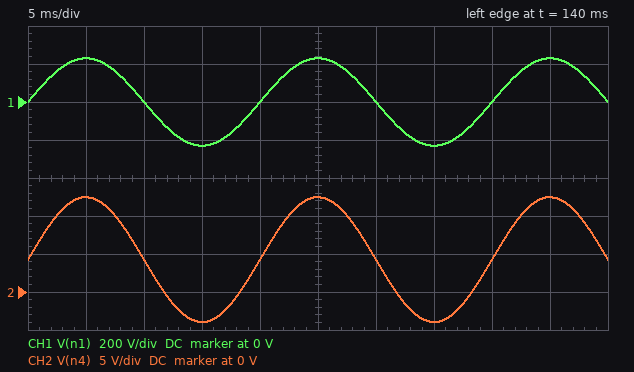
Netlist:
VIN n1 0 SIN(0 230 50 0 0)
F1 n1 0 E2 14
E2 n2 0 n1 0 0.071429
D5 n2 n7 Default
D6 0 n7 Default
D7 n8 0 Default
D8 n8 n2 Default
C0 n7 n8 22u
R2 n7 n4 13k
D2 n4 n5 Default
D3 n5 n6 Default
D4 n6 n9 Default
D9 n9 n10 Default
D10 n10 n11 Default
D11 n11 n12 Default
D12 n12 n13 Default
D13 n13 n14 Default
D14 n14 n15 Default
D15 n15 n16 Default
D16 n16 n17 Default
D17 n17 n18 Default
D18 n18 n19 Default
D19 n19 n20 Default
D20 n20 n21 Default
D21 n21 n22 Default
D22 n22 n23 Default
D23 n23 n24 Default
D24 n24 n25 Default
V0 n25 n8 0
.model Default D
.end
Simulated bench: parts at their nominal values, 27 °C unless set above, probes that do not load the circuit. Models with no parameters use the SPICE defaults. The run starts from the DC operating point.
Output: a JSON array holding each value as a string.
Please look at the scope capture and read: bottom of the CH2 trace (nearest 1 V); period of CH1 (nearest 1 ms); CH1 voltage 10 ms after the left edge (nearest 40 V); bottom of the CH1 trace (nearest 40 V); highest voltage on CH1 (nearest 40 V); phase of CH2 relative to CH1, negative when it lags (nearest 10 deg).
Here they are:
["-4 V", "20 ms", "0 V", "-240 V", "240 V", "0 deg"]
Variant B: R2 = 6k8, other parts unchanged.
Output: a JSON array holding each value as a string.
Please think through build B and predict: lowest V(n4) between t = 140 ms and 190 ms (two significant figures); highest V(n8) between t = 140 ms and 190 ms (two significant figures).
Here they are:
["-3.7 V", "710 mV"]
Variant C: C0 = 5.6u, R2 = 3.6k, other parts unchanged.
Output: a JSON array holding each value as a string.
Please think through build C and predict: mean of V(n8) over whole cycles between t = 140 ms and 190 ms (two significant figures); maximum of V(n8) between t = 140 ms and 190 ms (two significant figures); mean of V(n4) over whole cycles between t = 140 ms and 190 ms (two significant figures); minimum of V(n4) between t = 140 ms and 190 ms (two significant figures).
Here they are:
["-7.3 V", "710 mV", "4.9 V", "-3.4 V"]
